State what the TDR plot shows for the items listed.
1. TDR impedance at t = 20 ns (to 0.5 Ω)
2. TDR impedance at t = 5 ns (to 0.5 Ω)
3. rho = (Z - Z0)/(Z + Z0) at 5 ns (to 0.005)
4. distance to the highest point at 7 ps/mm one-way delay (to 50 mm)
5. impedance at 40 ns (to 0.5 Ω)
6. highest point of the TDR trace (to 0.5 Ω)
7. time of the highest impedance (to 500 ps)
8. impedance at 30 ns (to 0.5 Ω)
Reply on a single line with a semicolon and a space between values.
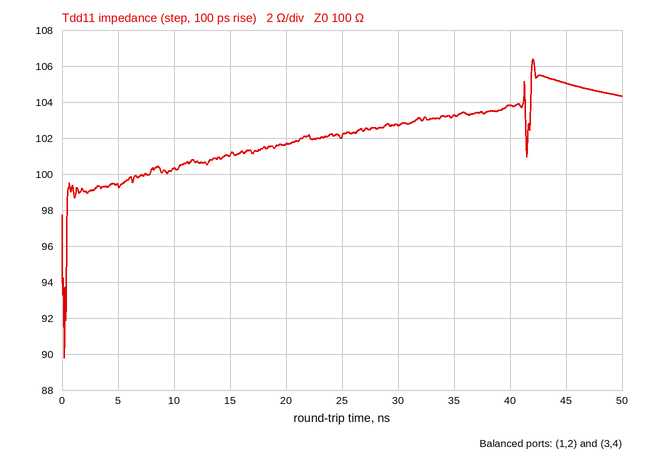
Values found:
101.5 Ω; 99.5 Ω; -0.005; 3.00 m; 104.0 Ω; 106.5 Ω; 42.0 ns; 102.5 Ω
